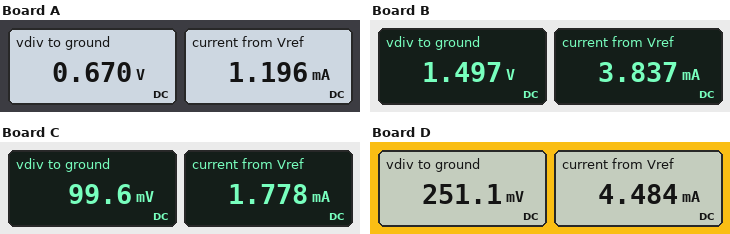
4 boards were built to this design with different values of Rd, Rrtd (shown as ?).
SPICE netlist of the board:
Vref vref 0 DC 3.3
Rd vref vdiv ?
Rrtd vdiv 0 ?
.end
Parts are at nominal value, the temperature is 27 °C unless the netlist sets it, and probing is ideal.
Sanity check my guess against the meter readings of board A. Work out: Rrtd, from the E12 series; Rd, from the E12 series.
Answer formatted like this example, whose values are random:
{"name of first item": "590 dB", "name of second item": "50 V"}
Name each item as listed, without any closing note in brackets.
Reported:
{"Rrtd, from the E12 series": "560 Ω", "Rd, from the E12 series": "2.2 kΩ"}
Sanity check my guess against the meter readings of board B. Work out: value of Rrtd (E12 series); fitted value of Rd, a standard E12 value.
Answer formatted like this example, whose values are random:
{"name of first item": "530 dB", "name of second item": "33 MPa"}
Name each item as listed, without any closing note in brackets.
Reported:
{"value of Rrtd": "390 Ω", "fitted value of Rd, a standard E12 value": "470 Ω"}
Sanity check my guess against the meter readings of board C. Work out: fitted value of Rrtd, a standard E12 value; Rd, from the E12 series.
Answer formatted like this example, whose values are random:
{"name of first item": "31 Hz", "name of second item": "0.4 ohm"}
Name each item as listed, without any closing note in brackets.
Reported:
{"fitted value of Rrtd, a standard E12 value": "56 Ω", "Rd, from the E12 series": "1.8 kΩ"}
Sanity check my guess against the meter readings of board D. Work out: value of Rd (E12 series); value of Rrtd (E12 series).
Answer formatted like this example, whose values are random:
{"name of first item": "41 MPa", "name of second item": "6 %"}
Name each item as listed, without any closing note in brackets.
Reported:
{"value of Rd": "680 Ω", "value of Rrtd": "56 Ω"}
